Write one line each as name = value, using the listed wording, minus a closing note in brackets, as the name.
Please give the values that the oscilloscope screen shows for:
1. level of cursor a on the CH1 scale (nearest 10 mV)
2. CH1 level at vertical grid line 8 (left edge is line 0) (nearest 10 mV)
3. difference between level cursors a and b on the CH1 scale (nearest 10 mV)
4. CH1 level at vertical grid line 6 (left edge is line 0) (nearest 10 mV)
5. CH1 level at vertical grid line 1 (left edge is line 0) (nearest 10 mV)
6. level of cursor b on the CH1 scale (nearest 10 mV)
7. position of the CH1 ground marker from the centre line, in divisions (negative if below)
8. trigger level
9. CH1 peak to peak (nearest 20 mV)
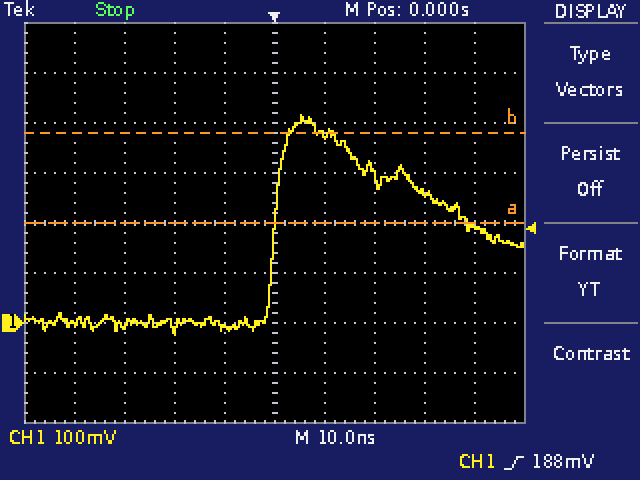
level of cursor a on the CH1 scale = 200 mV
CH1 level at vertical grid line 8 (left edge is line 0) = 260 mV
difference between level cursors a and b on the CH1 scale = 180 mV
CH1 level at vertical grid line 6 (left edge is line 0) = 380 mV
CH1 level at vertical grid line 1 (left edge is line 0) = 0 mV
level of cursor b on the CH1 scale = 380 mV
position of the CH1 ground marker from the centre line, in divisions = -2.0 div
trigger level = 188 mV
CH1 peak to peak = 440 mV
